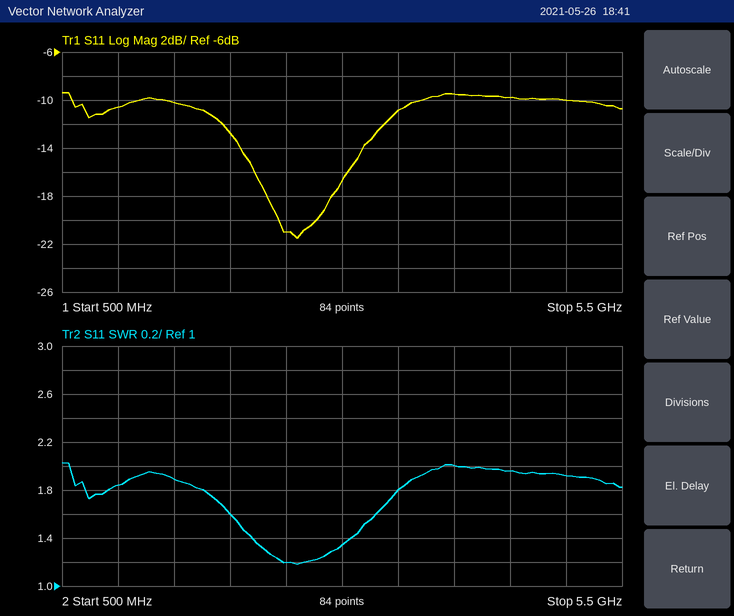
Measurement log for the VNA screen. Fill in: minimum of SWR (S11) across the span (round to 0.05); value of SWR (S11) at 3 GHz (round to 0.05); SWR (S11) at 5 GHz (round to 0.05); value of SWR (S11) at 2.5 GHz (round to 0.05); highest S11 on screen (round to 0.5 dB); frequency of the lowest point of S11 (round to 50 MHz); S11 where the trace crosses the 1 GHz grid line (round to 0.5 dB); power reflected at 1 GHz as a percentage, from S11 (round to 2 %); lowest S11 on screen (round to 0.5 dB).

1.20
1.35
1.90
1.20
-9.5 dB
2.60 GHz
-10.5 dB
8 %
-21.5 dB
